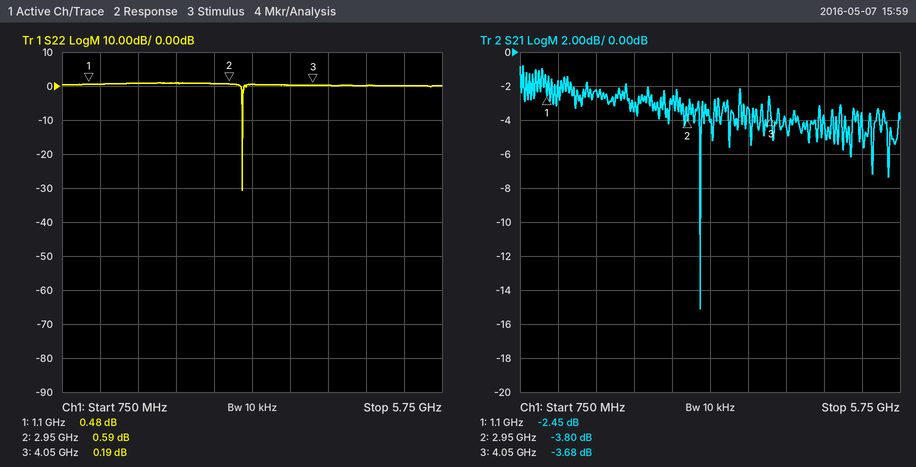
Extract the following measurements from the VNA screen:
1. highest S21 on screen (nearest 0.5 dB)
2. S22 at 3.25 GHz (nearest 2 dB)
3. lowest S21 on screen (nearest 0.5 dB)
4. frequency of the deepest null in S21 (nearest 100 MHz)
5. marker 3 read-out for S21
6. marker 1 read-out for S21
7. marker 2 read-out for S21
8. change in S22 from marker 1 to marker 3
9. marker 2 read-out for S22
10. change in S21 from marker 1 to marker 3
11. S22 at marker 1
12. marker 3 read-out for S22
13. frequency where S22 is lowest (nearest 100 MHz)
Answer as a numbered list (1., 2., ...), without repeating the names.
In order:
1. -1.0 dB
2. 0 dB
3. -15.0 dB
4. 3.1 GHz
5. -3.68 dB
6. -2.45 dB
7. -3.80 dB
8. -0.29 dB
9. 0.59 dB
10. -1.23 dB
11. 0.48 dB
12. 0.19 dB
13. 3.1 GHz
